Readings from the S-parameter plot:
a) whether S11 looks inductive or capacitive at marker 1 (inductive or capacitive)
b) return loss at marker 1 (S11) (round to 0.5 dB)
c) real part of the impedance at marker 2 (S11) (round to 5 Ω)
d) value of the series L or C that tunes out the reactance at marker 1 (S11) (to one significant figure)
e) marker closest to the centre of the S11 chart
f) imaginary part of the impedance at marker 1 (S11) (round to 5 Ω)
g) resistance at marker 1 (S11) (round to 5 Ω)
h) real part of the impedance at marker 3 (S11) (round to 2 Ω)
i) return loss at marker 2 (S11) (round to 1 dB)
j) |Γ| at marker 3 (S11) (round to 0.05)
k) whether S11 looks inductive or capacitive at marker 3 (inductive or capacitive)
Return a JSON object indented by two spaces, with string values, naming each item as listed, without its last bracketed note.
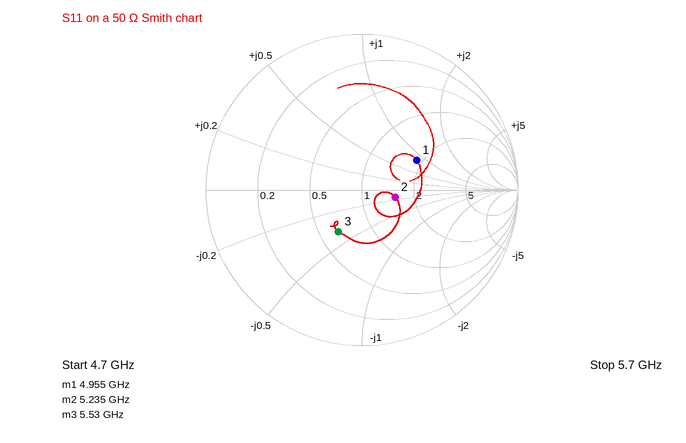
{
  "whether S11 looks inductive or capacitive at marker 1": "inductive",
  "return loss at marker 1 (S11)": "8.0 dB",
  "real part of the impedance at marker 2 (S11)": "75 Ω",
  "value of the series L or C that tunes out the reactance at marker 1 (S11)": "800 fF",
  "marker closest to the centre of the S11 chart": "marker 2",
  "imaginary part of the impedance at marker 1 (S11)": "+40 Ω",
  "resistance at marker 1 (S11)": "90 Ω",
  "real part of the impedance at marker 3 (S11)": "32 Ω",
  "return loss at marker 2 (S11)": "13 dB",
  "|Γ| at marker 3 (S11)": "0.30",
  "whether S11 looks inductive or capacitive at marker 3": "capacitive"
}
